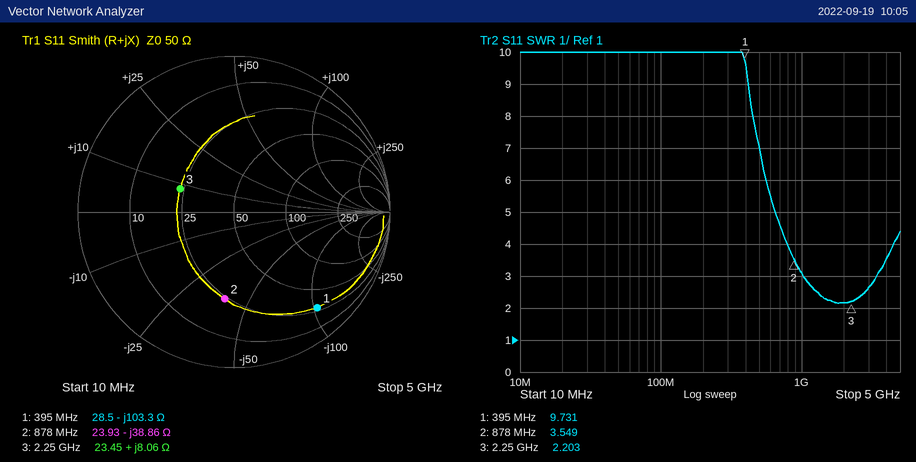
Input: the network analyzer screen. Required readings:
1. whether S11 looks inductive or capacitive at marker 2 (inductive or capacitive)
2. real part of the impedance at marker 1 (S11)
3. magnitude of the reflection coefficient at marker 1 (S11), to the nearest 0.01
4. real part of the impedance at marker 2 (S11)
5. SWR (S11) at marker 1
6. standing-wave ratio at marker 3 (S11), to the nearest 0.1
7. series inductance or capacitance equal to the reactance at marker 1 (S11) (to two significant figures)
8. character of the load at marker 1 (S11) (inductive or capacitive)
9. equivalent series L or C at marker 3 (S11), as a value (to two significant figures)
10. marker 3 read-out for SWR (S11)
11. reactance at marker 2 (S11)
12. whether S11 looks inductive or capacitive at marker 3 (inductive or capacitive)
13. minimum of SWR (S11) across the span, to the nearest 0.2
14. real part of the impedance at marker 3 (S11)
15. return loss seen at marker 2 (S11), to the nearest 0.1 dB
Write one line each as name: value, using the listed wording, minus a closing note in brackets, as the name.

whether S11 looks inductive or capacitive at marker 2: capacitive
real part of the impedance at marker 1: 28.5 Ω
magnitude of the reflection coefficient at marker 1 (S11), to the nearest 0.01: 0.81
real part of the impedance at marker 2: 23.93 Ω
SWR (S11) at marker 1: 9.731
standing-wave ratio at marker 3 (S11), to the nearest 0.1: 2.2
series inductance or capacitance equal to the reactance at marker 1 (S11): 3.9 pF
character of the load at marker 1 (S11): capacitive
equivalent series L or C at marker 3 (S11), as a value: 570 pH
marker 3 read-out for SWR: 2.203
reactance at marker 2: -38.86 Ω
whether S11 looks inductive or capacitive at marker 3: inductive
minimum of SWR (S11) across the span, to the nearest 0.2: 2.2
real part of the impedance at marker 3: 23.45 Ω
return loss seen at marker 2 (S11), to the nearest 0.1 dB: 5.0 dB
